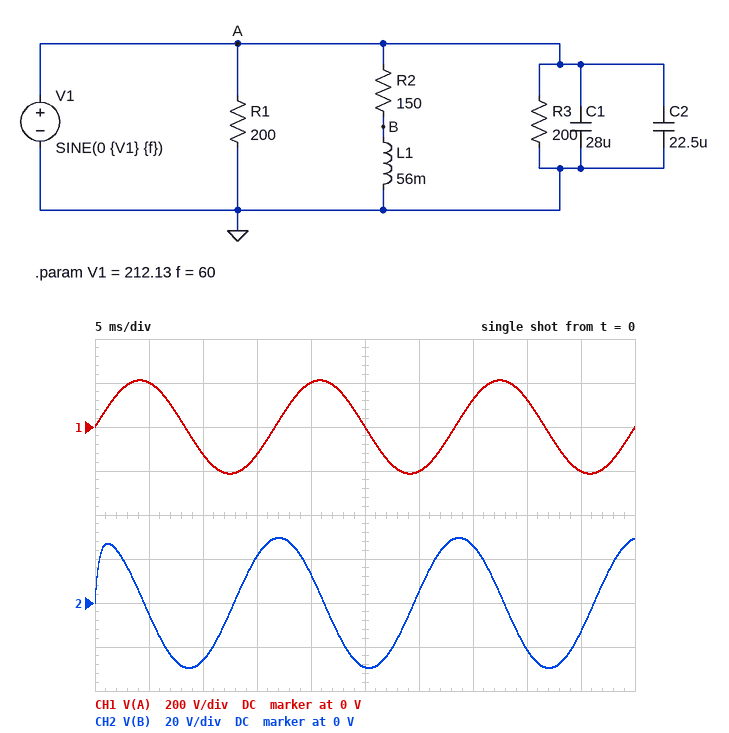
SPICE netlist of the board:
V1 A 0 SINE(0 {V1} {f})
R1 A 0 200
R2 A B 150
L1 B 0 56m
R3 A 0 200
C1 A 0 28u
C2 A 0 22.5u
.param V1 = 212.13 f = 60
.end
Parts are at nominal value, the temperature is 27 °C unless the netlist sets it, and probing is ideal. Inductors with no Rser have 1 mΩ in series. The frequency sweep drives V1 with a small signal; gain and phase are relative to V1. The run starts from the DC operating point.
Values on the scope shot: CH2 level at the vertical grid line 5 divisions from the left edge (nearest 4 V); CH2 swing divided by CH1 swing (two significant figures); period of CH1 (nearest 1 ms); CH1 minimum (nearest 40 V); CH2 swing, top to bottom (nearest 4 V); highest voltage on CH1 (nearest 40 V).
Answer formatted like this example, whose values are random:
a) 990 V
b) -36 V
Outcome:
a) -28 V
b) 0.14
c) 17 ms
d) -200 V
e) 60 V
f) 200 V
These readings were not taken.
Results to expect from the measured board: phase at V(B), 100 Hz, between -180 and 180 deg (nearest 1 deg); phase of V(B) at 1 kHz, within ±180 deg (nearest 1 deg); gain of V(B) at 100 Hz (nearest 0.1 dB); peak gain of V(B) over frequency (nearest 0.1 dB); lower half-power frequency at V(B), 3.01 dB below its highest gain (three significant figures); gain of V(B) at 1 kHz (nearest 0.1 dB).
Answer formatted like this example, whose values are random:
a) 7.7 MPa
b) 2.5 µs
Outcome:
a) 77 deg
b) 23 deg
c) -12.8 dB
d) 0 dB
e) 426 Hz
f) -0.7 dB
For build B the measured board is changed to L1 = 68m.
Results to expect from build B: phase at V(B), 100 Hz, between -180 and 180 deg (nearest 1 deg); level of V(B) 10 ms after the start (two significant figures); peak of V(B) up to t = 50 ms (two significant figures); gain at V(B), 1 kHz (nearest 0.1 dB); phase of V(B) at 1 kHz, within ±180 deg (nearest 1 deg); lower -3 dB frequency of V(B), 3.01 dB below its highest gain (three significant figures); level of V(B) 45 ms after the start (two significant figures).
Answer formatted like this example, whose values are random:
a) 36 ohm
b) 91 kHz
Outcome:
a) 74 deg
b) -32 V
c) 36 V
d) -0.5 dB
e) 19 deg
f) 351 Hz
g) -17 V
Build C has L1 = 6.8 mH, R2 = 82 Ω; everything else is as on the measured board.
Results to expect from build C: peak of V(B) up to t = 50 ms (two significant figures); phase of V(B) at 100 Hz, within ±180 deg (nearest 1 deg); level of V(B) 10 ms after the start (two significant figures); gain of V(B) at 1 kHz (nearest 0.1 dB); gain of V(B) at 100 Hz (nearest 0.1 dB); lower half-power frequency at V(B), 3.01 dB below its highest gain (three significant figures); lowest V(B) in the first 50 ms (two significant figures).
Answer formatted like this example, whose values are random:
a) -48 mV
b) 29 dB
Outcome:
a) 6.6 V
b) 87 deg
c) -5.5 V
d) -6.7 dB
e) -25.7 dB
f) 1.92 kHz
g) -6.6 V
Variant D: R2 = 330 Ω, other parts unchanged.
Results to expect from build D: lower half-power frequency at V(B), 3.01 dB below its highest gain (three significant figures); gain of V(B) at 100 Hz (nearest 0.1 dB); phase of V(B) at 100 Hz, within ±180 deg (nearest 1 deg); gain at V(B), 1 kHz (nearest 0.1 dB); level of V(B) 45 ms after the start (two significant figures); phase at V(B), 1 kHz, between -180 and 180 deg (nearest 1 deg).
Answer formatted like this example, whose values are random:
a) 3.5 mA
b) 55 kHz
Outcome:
a) 938 Hz
b) -19.5 dB
c) 84 deg
d) -2.7 dB
e) -5.0 V
f) 43 deg
